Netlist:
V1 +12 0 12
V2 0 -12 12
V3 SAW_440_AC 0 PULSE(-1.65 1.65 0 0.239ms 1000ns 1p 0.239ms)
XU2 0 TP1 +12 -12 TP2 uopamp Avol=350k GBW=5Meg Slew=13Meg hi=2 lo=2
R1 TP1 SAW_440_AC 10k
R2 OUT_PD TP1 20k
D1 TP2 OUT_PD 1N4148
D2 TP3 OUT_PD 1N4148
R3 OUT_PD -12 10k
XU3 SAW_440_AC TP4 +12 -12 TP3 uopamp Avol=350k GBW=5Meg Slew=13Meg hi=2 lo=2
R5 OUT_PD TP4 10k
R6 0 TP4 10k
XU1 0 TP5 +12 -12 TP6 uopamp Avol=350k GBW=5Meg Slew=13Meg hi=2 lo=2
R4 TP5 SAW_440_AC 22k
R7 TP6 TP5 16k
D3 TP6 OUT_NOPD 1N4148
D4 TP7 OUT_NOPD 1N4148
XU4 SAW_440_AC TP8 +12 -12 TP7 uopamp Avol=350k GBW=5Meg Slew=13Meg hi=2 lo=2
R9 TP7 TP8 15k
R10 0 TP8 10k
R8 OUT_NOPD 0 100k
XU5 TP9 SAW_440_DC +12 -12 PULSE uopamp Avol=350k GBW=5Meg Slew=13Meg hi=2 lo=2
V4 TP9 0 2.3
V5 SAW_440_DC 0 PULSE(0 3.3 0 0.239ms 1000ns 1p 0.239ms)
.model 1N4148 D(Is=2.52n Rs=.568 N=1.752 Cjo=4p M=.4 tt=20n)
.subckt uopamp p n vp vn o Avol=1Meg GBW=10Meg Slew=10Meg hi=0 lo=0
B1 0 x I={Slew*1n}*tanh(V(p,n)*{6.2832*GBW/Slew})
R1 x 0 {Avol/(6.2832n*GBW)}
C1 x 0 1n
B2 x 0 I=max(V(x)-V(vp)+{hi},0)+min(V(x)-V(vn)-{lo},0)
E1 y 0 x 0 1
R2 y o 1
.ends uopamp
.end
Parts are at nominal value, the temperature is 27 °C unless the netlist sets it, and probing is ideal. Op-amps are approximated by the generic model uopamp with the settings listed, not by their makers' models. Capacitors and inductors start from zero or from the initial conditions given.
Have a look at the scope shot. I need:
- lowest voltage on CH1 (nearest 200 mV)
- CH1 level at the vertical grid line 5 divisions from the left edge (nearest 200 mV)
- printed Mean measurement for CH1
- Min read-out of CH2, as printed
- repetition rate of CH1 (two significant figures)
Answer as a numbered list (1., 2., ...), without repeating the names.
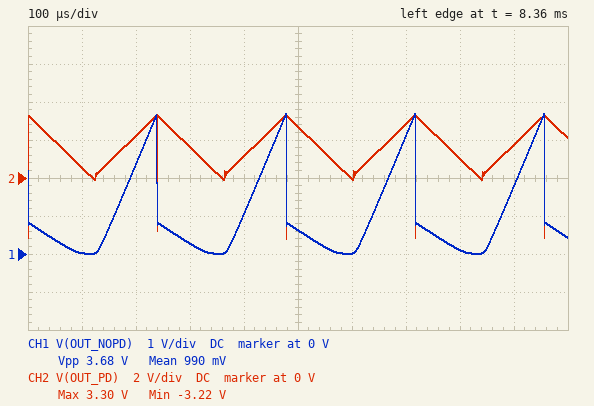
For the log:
1. 0 V
2. 600 mV
3. 990 mV
4. -3.22 V
5. 4.2 kHz
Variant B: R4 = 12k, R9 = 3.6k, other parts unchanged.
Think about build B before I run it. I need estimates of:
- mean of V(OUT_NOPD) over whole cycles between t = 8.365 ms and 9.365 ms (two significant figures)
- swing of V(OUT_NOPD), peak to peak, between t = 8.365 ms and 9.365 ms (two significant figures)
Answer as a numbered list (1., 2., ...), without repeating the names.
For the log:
1. 780 mV
2. 1.8 V
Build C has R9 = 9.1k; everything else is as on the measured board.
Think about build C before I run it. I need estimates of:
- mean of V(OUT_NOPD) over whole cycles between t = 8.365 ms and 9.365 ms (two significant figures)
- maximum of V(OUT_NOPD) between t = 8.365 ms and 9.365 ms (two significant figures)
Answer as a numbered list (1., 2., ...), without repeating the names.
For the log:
1. 770 mV
2. 2.7 V
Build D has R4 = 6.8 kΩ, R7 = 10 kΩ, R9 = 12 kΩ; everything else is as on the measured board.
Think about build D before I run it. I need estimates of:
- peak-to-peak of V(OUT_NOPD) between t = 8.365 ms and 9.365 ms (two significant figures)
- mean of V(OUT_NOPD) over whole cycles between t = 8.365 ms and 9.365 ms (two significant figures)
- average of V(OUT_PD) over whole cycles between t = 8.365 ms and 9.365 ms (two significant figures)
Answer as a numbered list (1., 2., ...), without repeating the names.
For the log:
1. 3.2 V
2. 1.2 V
3. 1.6 V
